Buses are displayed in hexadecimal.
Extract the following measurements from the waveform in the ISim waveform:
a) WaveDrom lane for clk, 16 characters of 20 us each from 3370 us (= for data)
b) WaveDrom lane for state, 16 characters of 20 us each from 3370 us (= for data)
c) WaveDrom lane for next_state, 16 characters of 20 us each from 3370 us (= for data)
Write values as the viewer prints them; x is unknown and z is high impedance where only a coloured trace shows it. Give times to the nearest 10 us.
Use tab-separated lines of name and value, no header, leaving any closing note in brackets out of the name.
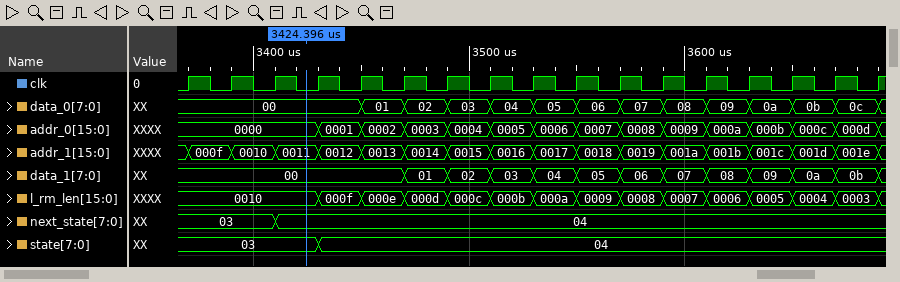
WaveDrom lane for clk, 16 characters of 20 us each from 3370 us	{name: 'clk', wave: 'p...............'}
WaveDrom lane for state, 16 characters of 20 us each from 3370 us	{name: 'state', wave: '=..=............', data: '03 04'}
WaveDrom lane for next_state, 16 characters of 20 us each from 3370 us	{name: 'next_state', wave: '=.=.............', data: '03 04'}
